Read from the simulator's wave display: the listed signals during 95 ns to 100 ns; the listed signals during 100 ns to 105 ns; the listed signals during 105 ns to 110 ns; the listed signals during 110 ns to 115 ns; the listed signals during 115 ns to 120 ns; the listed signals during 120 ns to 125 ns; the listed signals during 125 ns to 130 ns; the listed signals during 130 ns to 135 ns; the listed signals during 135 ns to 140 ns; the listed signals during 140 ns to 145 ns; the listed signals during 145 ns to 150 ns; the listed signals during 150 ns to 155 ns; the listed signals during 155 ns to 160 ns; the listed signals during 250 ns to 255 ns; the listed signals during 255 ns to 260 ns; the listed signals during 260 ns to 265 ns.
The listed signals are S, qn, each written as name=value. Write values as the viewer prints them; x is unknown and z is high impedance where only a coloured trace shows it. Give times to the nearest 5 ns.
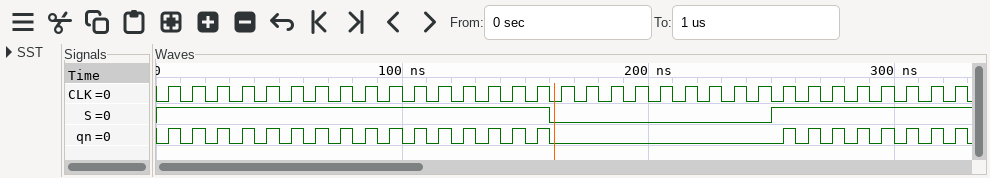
S=1, qn=1
S=1, qn=0
S=1, qn=1
S=1, qn=0
S=1, qn=1
S=1, qn=0
S=1, qn=1
S=1, qn=0
S=1, qn=1
S=1, qn=0
S=1, qn=1
S=1, qn=0
S=1, qn=1
S=1, qn=0
S=1, qn=1
S=1, qn=0
